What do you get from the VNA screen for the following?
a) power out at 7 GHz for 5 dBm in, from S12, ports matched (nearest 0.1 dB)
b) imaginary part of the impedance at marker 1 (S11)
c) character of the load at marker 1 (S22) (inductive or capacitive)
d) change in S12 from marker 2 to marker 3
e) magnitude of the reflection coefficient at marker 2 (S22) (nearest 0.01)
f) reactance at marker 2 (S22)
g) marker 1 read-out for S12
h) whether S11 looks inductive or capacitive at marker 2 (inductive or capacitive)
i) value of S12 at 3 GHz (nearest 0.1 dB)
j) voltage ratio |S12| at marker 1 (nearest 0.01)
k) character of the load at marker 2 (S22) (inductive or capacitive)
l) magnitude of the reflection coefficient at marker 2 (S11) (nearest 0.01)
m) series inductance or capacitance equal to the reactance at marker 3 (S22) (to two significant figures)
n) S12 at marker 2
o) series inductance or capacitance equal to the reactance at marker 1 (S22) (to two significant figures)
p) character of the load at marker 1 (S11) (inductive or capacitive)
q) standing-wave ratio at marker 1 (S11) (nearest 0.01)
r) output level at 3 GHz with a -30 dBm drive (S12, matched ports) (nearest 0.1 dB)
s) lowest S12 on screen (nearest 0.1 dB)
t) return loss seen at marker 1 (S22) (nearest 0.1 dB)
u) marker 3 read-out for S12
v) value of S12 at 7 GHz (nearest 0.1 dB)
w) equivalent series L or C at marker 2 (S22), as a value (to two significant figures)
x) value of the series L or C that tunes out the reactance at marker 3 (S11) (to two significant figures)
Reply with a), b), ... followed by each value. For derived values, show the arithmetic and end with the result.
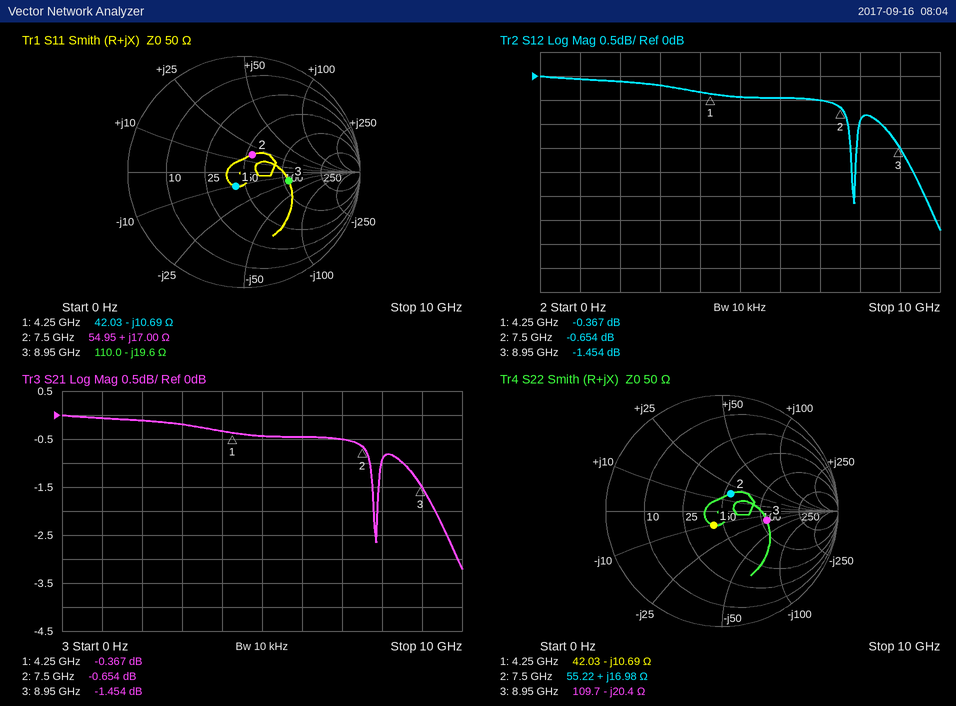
a) 5 dBm + (-0.5 dB) = 4.5 dBm
b) -10.69 Ω
c) capacitive
d) -1.454 − (-0.654) = -0.800 dB
e) 0.17
f) +16.98 Ω
g) -0.367 dB
h) inductive
i) -0.2 dB
j) 10^(-0.367/20) ≈ 0.96
k) inductive
l) 0.17
m) C = 1/(2π × 8.95 GHz × 20.4 Ω) ≈ 872 fF, so 870 fF to two significant figures
n) -0.654 dB
o) C = 1/(2π × 4.25 GHz × 10.69 Ω) ≈ 3.5 pF
p) capacitive
q) 1.34
r) -30 dBm + (-0.2 dB) = -30.2 dBm
s) -3.2 dB
t) 16.8 dB
u) -1.454 dB
v) -0.5 dB
w) L = 16.98 Ω/(2π × 7.5 GHz) ≈ 360 pH
x) L = 19.6 Ω/(2π × 8.95 GHz) ≈ 349 pH, so 350 pH to two significant figures
